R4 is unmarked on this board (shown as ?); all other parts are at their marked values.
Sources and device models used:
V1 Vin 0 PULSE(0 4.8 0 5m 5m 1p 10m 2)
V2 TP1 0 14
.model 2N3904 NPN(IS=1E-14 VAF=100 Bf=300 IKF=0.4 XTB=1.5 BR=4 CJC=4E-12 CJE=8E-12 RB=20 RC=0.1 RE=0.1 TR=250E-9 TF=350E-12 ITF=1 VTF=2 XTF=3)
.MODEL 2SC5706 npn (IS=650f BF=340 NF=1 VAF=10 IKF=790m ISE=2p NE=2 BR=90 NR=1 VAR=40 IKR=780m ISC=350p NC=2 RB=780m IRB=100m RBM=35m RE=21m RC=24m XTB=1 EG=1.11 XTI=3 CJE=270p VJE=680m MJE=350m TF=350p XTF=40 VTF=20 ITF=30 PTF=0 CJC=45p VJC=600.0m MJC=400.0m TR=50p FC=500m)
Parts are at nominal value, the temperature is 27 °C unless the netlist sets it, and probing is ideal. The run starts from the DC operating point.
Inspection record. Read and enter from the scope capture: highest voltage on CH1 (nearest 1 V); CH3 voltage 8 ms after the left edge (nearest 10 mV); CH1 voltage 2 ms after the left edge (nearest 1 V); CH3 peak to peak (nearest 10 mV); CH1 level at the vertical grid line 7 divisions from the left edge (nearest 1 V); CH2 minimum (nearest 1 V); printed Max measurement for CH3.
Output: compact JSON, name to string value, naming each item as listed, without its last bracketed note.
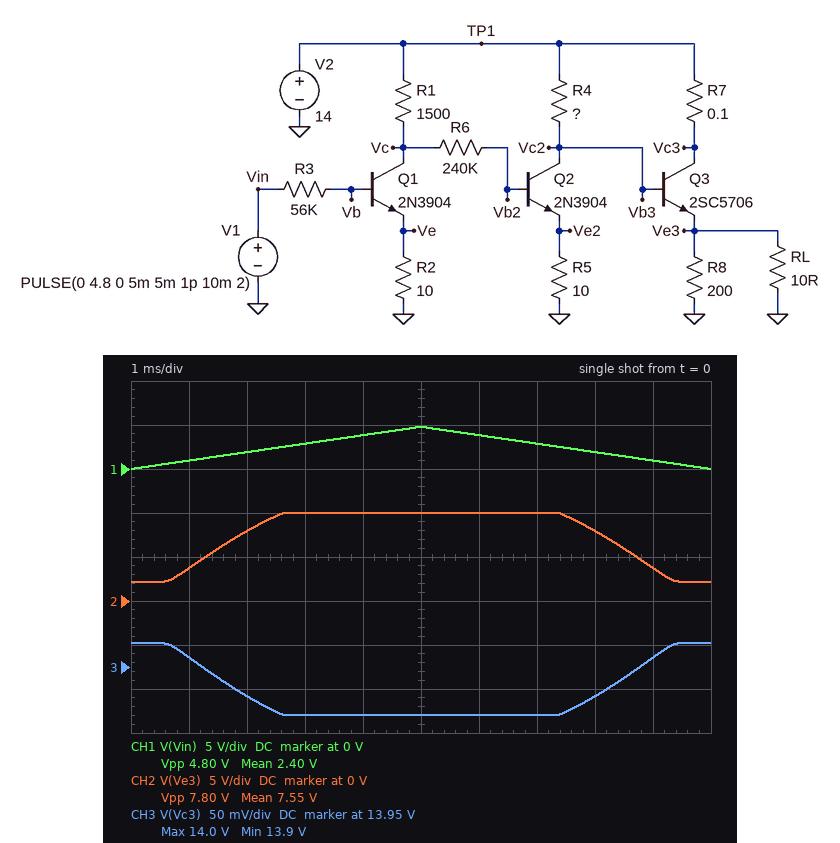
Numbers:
{"highest voltage on CH1": "5 V", "CH3 voltage 8 ms after the left edge": "13.92 V", "CH1 voltage 2 ms after the left edge": "2 V", "CH3 peak to peak": "80 mV", "CH1 level at the vertical grid line 7 divisions from the left edge": "3 V", "CH2 minimum": "2 V", "printed Max measurement for CH3": "14.0 V"}
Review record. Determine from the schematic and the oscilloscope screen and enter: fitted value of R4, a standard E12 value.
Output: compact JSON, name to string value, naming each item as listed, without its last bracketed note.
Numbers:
{"fitted value of R4, a standard E12 value": "680 Ω"}
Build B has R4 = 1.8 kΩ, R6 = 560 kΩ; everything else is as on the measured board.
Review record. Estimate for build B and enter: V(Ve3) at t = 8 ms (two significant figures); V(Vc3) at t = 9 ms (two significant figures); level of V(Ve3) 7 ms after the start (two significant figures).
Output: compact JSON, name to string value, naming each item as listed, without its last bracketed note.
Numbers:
{"V(Ve3) at t = 8 ms": "6.3 V", "V(Vc3) at t = 9 ms": "14 V", "level of V(Ve3) 7 ms after the start": "8.1 V"}
